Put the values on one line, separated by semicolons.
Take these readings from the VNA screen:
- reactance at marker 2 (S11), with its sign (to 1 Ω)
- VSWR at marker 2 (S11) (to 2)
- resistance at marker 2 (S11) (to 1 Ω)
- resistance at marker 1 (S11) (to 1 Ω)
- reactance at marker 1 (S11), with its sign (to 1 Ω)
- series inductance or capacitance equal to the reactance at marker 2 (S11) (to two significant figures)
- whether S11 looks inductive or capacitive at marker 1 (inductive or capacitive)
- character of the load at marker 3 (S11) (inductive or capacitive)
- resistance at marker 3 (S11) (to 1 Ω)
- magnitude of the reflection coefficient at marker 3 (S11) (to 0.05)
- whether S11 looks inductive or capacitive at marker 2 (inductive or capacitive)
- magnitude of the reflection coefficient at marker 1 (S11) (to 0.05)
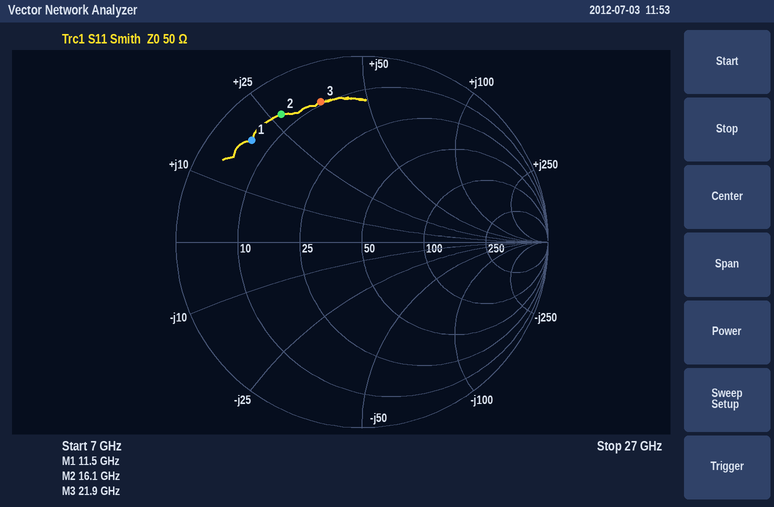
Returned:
+27 Ω; 10; 7 Ω; 6 Ω; +19 Ω; 270 pH; inductive; inductive; 9 Ω; 0.80; inductive; 0.80
